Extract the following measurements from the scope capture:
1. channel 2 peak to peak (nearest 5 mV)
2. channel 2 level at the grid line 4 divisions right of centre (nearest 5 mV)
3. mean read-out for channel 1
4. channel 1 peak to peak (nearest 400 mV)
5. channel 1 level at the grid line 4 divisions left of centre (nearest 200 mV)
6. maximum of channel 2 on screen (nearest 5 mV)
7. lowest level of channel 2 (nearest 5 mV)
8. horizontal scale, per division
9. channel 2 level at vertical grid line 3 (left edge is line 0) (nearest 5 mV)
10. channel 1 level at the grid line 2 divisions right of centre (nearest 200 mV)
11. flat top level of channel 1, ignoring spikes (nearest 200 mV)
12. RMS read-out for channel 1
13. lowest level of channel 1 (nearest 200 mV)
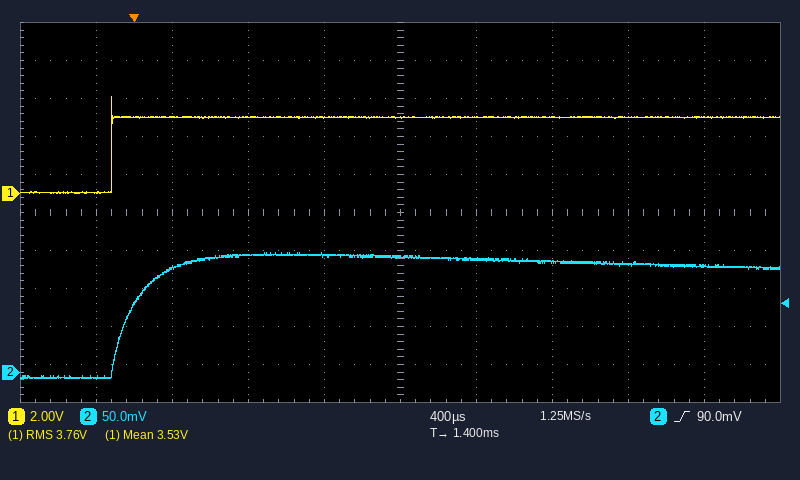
165 mV
140 mV
3.53 V
5.2 V
0.0 V
155 mV
-10 mV
400 µs
155 mV
4.0 V
4.0 V
3.76 V
0.0 V
